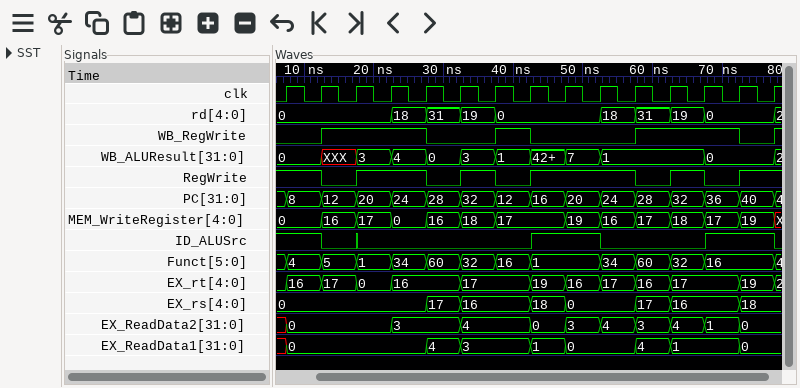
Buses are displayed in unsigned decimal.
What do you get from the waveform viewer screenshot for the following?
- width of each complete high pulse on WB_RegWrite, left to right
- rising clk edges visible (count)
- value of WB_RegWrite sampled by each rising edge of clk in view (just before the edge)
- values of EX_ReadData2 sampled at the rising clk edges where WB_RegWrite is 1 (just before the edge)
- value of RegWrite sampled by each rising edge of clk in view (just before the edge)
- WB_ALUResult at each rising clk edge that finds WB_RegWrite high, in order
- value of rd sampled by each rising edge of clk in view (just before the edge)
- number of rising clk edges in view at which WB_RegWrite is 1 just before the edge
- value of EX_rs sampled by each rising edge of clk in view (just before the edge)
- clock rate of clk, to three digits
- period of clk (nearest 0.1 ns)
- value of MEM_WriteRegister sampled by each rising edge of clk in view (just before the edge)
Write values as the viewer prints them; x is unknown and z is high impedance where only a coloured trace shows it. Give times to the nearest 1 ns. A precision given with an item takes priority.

15 ns, 5 ns, 15 ns
15
0 0 1 1 1 0 0 1 0 0 0 1 1 1 0
0, 0, 3, 4, 3, 4, 1
1 1 0 1 1 0 1 0 1 1 1 0 1 0 1
XXX, 3, 4, 1, 1, 1, 0
0, 0, 0, 0, 18, 31, 19, 0, 0, 0, 18, 31, 19, 0, 0
7
0, 0, 0, 0, 0, 17, 16, 16, 18, 0, 0, 17, 16, 16, 18
200 MHz
5 ns
0, 0, 16, 17, 0, 16, 18, 17, 17, 19, 16, 17, 18, 17, 19
